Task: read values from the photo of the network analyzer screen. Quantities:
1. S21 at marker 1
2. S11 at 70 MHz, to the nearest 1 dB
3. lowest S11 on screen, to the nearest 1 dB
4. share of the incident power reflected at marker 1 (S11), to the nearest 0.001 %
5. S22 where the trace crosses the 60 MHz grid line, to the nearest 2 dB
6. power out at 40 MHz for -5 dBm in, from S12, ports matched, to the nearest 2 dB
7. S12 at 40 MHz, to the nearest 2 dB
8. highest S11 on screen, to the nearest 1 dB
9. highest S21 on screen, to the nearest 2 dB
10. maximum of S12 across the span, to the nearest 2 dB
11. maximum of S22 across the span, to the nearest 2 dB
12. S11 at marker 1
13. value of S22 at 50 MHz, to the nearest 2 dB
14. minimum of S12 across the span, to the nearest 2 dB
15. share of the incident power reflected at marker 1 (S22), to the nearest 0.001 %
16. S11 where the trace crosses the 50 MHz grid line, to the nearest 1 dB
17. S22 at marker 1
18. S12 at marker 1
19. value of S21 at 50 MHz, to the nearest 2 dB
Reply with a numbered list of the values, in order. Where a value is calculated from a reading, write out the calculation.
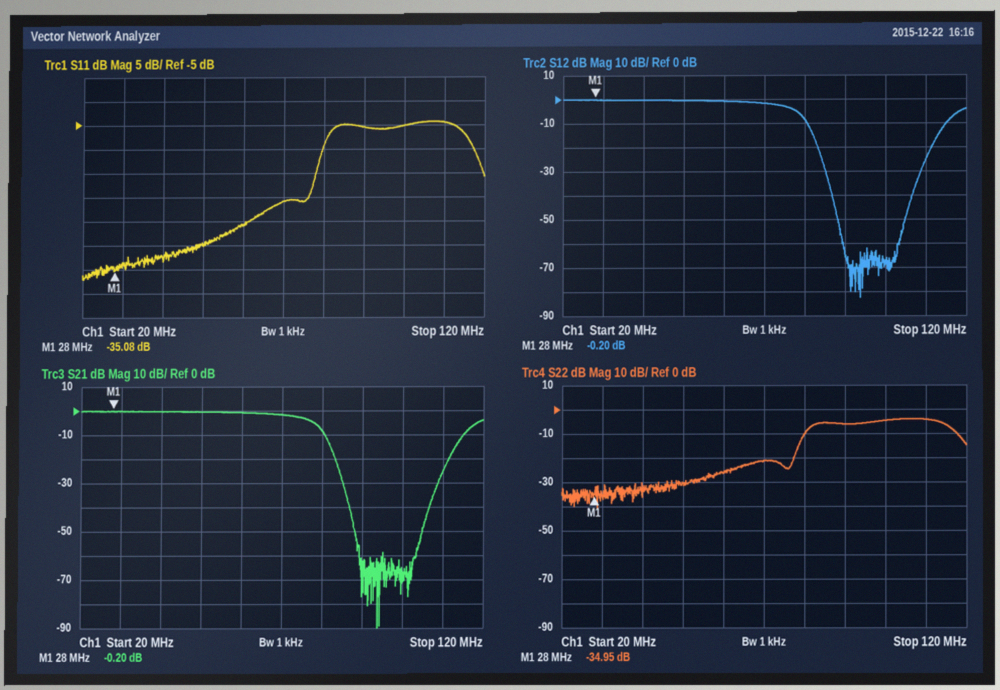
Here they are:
1. -0.20 dB
2. -21 dB
3. -37 dB
4. 10^(-35.08/10) ≈ 0.031 %
5. -26 dB
6. -5 dBm + (0 dB) = -6 dBm
7. 0 dB
8. -4 dB
9. 0 dB
10. 0 dB
11. -4 dB
12. -35.08 dB
13. -30 dB
14. -82 dB
15. 10^(-34.95/10) ≈ 0.032 %
16. -30 dB
17. -34.95 dB
18. -0.20 dB
19. 0 dB
